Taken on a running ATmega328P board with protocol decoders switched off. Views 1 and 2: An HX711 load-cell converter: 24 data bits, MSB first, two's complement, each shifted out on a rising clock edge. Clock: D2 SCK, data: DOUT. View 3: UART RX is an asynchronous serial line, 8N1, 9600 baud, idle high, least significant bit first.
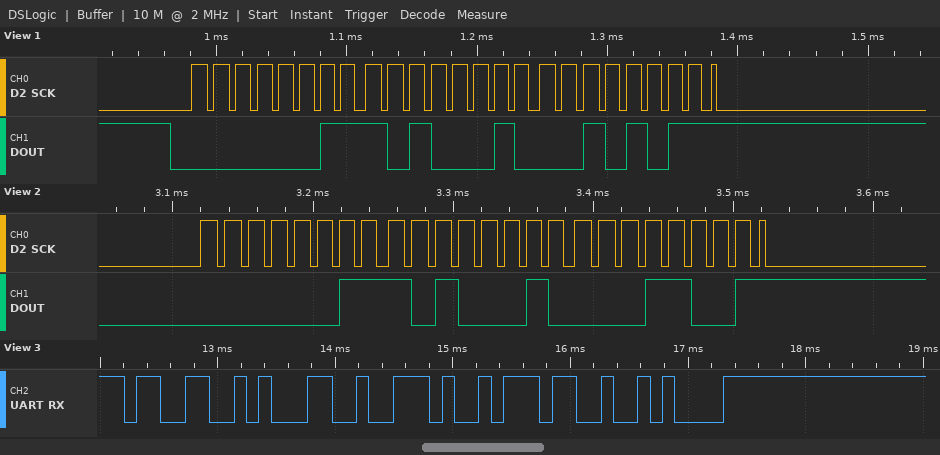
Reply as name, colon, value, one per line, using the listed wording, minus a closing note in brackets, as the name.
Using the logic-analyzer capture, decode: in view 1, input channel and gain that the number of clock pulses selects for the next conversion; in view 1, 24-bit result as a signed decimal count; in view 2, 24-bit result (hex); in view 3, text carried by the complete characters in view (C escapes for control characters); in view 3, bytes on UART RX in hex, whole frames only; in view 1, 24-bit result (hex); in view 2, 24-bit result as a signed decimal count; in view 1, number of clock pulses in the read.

in view 1, input channel and gain that the number of clock pulses selects for the next conversion: channel A, gain 128
in view 1, 24-bit result as a signed decimal count: 238123
in view 2, 24-bit result: 0x03A219
in view 3, text carried by the complete characters in view: "31.7\n"
in view 3, bytes on UART RX in hex, whole frames only: 33 31 2E 37 0A
in view 1, 24-bit result: 0x03A22B
in view 2, 24-bit result as a signed decimal count: 238105
in view 1, number of clock pulses in the read: 25
